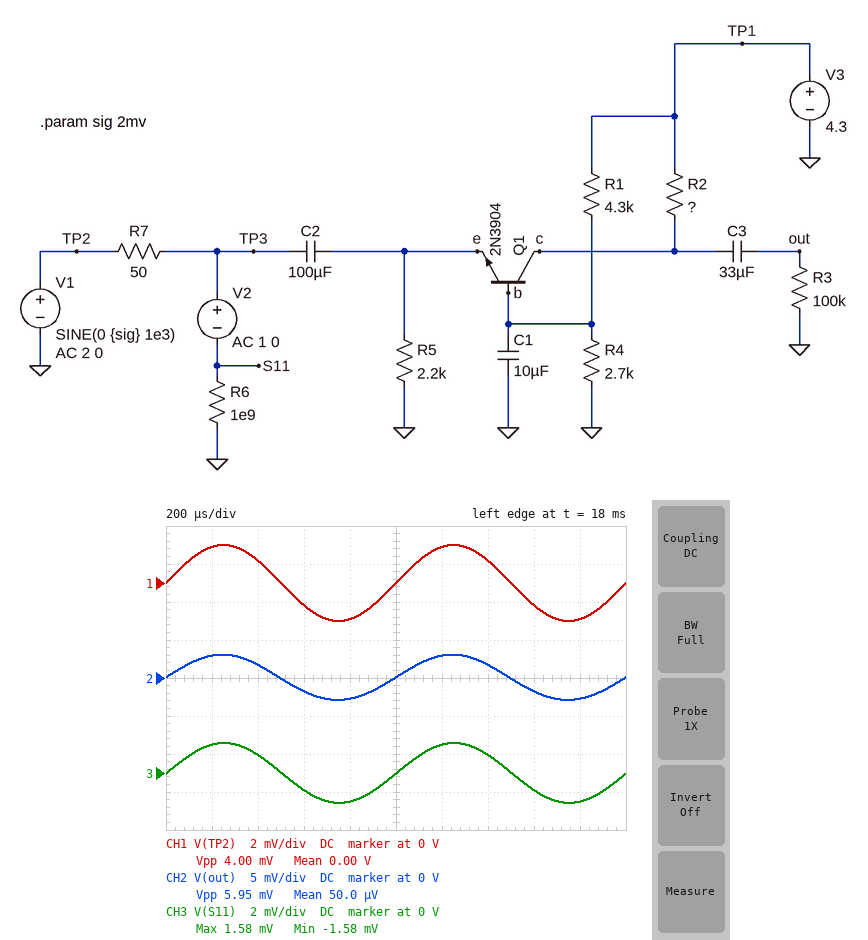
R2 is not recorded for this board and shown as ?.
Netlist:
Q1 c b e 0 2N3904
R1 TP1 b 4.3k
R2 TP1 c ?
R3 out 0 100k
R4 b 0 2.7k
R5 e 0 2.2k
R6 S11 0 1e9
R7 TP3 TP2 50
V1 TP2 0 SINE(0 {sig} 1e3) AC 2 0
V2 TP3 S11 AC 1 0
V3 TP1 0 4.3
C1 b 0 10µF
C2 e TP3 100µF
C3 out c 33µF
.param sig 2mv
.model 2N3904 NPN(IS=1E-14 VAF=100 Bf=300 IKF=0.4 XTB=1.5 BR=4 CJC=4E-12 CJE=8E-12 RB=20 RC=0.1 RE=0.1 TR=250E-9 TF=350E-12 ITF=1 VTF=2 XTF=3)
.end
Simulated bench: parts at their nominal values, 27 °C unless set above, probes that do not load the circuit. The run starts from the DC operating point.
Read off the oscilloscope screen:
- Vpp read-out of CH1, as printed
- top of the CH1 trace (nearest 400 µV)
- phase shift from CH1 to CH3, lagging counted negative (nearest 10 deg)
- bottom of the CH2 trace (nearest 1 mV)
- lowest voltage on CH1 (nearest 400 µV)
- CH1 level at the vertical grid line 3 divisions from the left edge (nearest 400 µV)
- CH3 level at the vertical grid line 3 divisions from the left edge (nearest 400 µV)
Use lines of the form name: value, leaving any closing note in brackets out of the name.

Vpp read-out of CH1, as printed: 4.00 mV
top of the CH1 trace: 2.0 mV
phase shift from CH1 to CH3, lagging counted negative: 0 deg
bottom of the CH2 trace: -3 mV
lowest voltage on CH1: -2.0 mV
CH1 level at the vertical grid line 3 divisions from the left edge: -1.2 mV
CH3 level at the vertical grid line 3 divisions from the left edge: -800 µV
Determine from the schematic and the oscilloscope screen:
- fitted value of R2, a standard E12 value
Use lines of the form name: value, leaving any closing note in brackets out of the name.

fitted value of R2, a standard E12 value: 10 kΩ
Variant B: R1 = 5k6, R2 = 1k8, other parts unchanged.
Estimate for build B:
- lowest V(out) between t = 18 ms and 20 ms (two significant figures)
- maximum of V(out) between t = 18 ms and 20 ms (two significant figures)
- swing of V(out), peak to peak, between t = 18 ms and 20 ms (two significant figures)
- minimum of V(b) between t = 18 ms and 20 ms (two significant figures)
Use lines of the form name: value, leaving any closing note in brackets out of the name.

lowest V(out) between t = 18 ms and 20 ms: -28 mV
maximum of V(out) between t = 18 ms and 20 ms: 28 mV
swing of V(out), peak to peak, between t = 18 ms and 20 ms: 56 mV
minimum of V(b) between t = 18 ms and 20 ms: 1.4 V
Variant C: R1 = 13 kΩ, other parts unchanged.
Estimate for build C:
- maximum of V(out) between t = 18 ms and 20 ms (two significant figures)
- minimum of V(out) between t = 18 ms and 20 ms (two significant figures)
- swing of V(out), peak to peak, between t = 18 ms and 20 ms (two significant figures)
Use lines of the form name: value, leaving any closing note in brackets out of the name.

maximum of V(out) between t = 18 ms and 20 ms: 41 mV
minimum of V(out) between t = 18 ms and 20 ms: -43 mV
swing of V(out), peak to peak, between t = 18 ms and 20 ms: 84 mV
